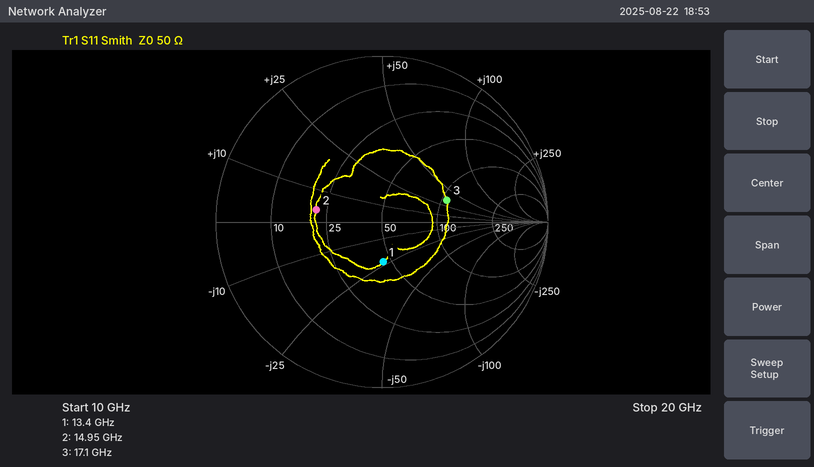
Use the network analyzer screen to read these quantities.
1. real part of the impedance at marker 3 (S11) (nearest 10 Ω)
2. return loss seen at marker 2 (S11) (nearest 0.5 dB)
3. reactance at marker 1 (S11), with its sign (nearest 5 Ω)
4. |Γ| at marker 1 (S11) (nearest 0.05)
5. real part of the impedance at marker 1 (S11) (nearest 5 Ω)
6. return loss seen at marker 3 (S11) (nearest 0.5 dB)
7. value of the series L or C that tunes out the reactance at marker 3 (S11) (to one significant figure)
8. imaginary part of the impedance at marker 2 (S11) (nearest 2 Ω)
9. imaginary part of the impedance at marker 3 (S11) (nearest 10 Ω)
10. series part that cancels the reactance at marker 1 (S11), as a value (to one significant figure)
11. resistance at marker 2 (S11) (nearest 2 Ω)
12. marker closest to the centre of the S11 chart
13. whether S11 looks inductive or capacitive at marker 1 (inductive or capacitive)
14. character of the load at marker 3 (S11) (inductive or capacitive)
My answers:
110 Ω
8.0 dB
-25 Ω
0.25
45 Ω
7.5 dB
300 fF
+4 Ω
+30 Ω
300 pH
22 Ω
marker 1
capacitive
inductive
